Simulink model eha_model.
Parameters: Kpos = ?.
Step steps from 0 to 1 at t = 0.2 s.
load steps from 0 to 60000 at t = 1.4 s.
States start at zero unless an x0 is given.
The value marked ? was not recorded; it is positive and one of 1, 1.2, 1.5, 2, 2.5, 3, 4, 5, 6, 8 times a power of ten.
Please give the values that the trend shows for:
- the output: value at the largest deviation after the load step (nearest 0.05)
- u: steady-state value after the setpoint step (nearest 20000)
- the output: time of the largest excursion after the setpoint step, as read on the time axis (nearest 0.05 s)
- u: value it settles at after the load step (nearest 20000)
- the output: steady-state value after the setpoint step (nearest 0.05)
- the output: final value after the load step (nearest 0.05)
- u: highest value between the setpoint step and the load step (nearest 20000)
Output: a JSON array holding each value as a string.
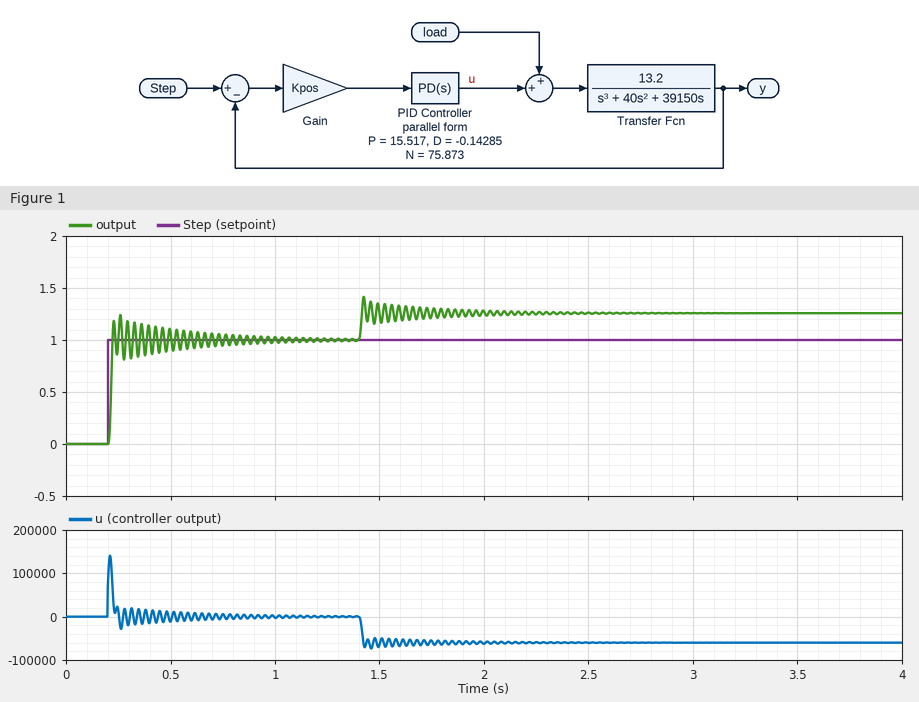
["1.40", "0", "0.25 s", "-60000", "1.00", "1.25", "140000"]
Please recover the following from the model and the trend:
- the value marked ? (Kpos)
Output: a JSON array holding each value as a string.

["15000"]
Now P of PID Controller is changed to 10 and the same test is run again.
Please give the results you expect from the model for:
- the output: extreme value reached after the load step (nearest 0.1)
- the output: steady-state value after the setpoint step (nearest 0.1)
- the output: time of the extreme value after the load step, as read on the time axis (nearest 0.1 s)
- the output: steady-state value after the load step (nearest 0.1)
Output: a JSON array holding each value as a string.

["1.5", "1.0", "1.4 s", "1.4"]
